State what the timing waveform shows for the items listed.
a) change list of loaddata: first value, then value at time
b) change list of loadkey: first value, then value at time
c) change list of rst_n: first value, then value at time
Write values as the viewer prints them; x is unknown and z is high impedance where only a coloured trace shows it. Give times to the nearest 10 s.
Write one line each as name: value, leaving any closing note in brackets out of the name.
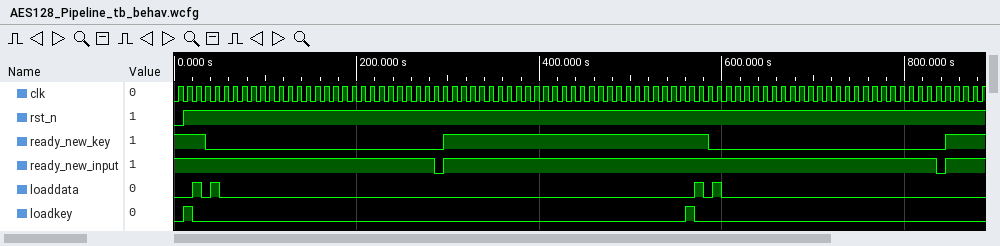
change list of loaddata: first value, then value at time: 0, 1 at 20 s, 0 at 30 s, 1 at 40 s, 0 at 50 s, 1 at 570 s, 0 at 580 s, 1 at 590 s, 0 at 600 s
change list of loadkey: first value, then value at time: 0, 1 at 10 s, 0 at 20 s, 1 at 560 s, 0 at 570 s
change list of rst_n: first value, then value at time: 0, 1 at 10 s
